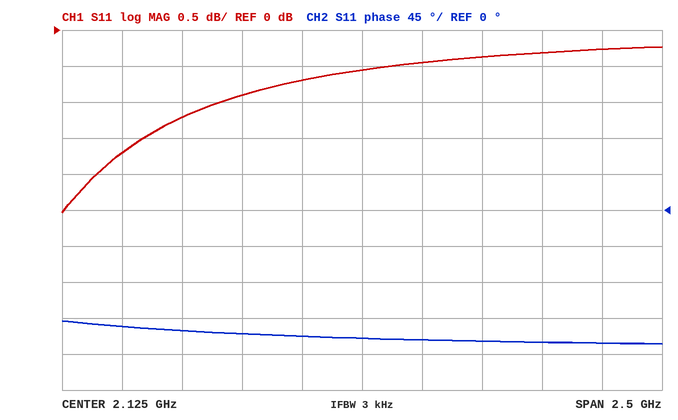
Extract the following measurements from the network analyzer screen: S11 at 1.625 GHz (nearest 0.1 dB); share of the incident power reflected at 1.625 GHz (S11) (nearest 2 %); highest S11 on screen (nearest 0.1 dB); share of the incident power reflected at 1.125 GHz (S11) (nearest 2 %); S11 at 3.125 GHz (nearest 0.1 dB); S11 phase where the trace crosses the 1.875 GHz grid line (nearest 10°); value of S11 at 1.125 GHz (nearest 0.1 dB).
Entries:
-0.9 dB
82 %
-0.2 dB
68 %
-0.3 dB
-160°
-1.7 dB
